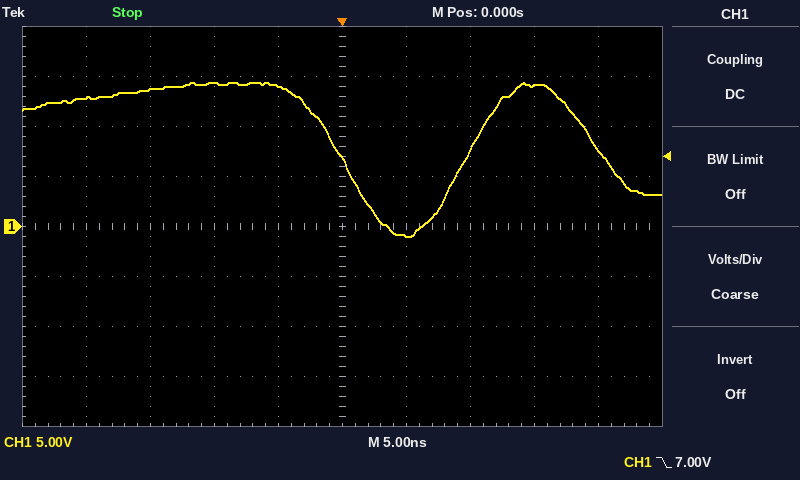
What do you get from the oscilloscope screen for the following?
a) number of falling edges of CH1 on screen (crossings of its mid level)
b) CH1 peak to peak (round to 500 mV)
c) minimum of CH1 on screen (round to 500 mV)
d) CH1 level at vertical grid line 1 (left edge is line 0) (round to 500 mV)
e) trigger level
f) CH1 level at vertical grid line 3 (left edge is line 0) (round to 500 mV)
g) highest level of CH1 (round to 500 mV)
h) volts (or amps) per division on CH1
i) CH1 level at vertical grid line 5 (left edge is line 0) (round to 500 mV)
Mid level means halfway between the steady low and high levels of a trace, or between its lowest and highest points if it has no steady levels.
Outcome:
2
15.5 V
-1.0 V
13.0 V
7.00 V
14.5 V
14.5 V
5 V
7.0 V
